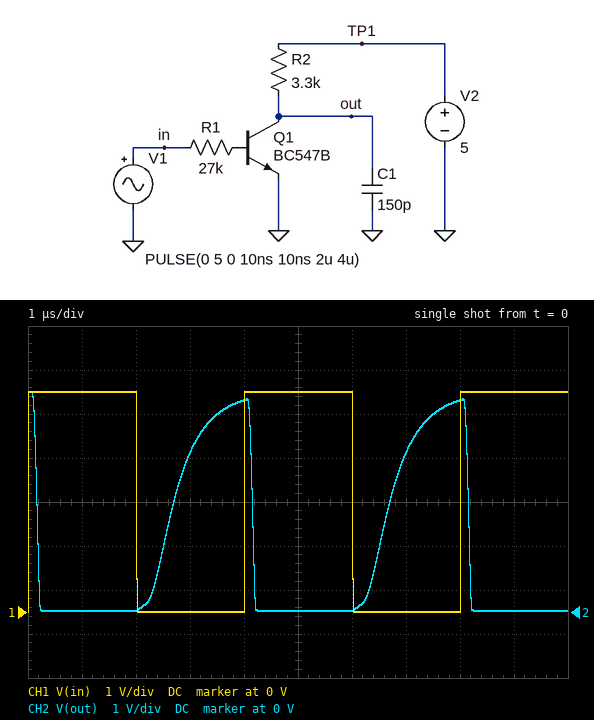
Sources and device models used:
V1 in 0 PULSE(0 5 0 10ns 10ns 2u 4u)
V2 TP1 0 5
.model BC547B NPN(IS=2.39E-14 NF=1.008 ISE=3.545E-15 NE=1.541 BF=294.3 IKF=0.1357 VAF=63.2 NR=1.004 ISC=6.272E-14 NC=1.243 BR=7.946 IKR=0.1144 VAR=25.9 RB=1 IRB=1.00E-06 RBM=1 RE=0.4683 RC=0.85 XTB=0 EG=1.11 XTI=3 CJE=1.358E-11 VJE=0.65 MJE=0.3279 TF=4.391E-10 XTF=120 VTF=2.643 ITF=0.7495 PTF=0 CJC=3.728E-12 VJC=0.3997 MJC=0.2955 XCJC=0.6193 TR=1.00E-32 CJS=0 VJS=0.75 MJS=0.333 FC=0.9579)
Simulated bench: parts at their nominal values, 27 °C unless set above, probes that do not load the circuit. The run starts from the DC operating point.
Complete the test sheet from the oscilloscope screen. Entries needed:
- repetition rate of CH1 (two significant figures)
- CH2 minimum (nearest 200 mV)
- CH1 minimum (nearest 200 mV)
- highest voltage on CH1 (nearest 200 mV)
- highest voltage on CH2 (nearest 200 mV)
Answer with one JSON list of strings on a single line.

["250 kHz", "0 V", "0 V", "5.0 V", "5.0 V"]
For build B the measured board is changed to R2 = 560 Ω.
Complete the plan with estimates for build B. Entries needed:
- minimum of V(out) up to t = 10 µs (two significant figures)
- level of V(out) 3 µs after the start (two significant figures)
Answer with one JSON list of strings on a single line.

["82 mV", "5.0 V"]
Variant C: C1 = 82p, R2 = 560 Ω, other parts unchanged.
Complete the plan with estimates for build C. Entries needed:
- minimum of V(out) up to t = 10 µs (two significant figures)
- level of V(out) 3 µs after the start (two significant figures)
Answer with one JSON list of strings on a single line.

["82 mV", "5.0 V"]
